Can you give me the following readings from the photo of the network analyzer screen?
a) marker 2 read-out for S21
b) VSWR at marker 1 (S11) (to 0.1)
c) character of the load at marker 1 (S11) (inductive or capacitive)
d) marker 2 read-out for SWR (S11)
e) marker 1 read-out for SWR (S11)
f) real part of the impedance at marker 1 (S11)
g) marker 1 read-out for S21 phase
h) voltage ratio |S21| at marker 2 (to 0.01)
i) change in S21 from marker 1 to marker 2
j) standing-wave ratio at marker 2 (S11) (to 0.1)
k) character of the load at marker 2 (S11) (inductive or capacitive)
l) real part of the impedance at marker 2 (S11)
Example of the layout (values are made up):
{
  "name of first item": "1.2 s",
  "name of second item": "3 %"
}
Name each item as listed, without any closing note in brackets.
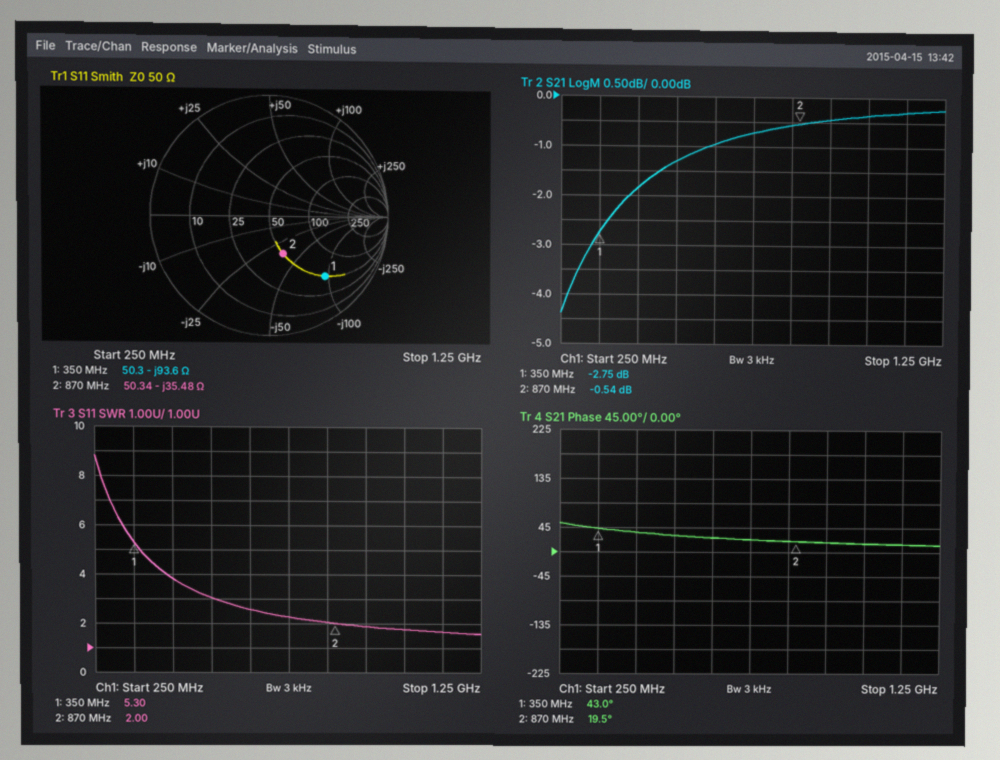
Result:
{
  "marker 2 read-out for S21": "-0.54 dB",
  "VSWR at marker 1 (S11)": "5.3",
  "character of the load at marker 1 (S11)": "capacitive",
  "marker 2 read-out for SWR": "2.00",
  "marker 1 read-out for SWR": "5.30",
  "real part of the impedance at marker 1": "50.3 Ω",
  "marker 1 read-out for S21 phase": "43.0°",
  "voltage ratio |S21| at marker 2": "0.94",
  "change in S21 from marker 1 to marker 2": "2.21 dB",
  "standing-wave ratio at marker 2 (S11)": "2.0",
  "character of the load at marker 2 (S11)": "capacitive",
  "real part of the impedance at marker 2": "50.34 Ω"
}
